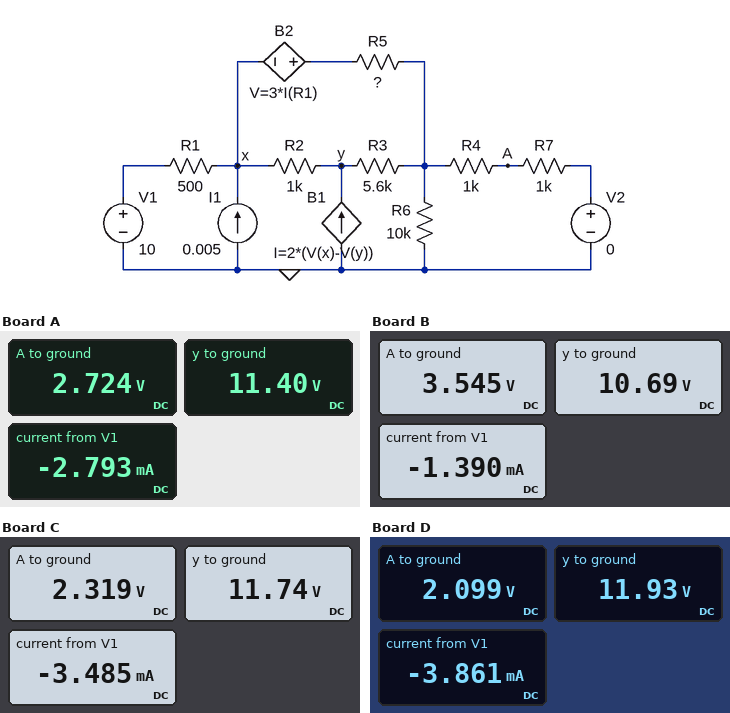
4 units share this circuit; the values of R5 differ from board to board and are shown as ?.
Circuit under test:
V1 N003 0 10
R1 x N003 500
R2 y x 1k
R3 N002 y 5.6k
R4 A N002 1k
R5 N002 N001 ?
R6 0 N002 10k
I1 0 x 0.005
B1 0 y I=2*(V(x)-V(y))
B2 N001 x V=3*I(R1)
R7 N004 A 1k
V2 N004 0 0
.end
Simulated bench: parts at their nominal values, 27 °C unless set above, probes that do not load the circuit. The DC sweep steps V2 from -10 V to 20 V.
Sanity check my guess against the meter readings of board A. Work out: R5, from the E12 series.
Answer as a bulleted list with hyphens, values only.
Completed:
- 2.7 kΩ
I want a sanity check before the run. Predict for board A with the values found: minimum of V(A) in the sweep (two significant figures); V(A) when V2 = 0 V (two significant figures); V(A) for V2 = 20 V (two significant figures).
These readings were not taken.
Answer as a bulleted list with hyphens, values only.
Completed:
- -4.6 V
- 2.7 V
- 17 V
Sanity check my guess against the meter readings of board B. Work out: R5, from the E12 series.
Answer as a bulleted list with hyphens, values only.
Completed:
- 1 kΩ
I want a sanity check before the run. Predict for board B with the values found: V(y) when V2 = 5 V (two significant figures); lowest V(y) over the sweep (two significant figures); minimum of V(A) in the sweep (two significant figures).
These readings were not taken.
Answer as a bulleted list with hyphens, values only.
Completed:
- 11 V
- 9.5 V
- -3.3 V
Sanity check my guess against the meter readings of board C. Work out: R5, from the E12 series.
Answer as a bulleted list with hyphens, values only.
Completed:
- 4.7 kΩ
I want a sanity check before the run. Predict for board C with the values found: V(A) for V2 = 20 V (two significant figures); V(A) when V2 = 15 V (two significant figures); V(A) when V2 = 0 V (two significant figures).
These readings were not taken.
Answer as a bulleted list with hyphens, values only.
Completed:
- 18 V
- 14 V
- 2.3 V
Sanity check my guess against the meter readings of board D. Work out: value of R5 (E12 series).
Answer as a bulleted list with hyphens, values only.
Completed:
- 6.8 kΩ
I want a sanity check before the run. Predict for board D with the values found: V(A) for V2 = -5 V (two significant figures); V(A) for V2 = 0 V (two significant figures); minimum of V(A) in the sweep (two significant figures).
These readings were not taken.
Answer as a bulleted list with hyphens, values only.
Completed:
- -1.8 V
- 2.1 V
- -5.7 V
